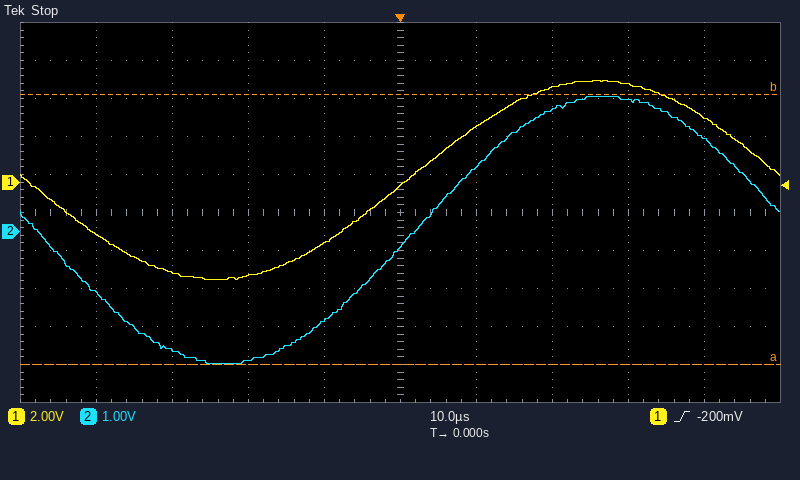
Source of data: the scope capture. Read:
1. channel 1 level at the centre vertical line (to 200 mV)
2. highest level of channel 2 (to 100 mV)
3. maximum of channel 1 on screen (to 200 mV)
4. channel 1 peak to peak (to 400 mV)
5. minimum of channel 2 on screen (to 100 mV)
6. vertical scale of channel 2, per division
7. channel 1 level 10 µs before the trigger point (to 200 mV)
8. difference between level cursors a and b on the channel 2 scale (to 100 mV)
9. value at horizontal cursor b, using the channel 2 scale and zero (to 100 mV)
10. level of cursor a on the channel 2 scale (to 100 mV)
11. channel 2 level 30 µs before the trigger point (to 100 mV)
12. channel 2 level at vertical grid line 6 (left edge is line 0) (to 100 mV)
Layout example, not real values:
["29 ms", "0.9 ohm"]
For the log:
["-200 mV", "3.6 V", "5.4 V", "10.4 V", "-3.5 V", "1 V", "-3.2 V", "7.1 V", "3.6 V", "-3.5 V", "-3.1 V", "1.7 V"]
